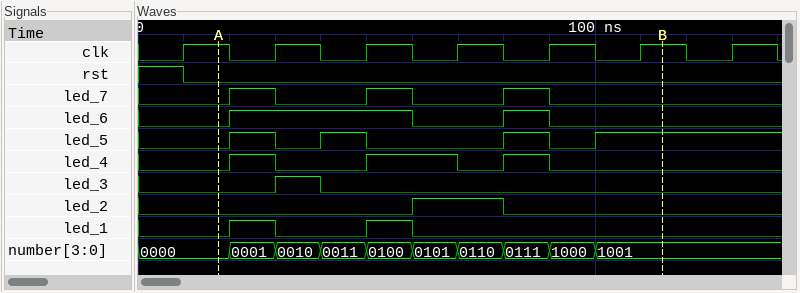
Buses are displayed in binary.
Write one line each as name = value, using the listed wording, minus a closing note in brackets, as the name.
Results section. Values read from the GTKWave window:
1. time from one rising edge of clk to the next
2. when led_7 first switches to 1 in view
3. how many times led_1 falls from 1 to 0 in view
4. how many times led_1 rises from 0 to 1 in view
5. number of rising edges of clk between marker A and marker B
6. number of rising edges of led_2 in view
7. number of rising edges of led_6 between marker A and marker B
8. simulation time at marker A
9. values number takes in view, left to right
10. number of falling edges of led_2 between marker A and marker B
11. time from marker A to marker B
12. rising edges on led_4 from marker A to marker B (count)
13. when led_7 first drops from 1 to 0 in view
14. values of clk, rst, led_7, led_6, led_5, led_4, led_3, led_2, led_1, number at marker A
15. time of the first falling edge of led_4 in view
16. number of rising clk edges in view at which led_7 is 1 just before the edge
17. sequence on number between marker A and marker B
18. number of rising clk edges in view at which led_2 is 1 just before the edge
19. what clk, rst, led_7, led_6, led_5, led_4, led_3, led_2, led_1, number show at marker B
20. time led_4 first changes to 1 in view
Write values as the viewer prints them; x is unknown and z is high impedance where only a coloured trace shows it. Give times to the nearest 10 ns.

time from one rising edge of clk to the next = 20 ns
when led_7 first switches to 1 in view = 20 ns
how many times led_1 falls from 1 to 0 in view = 2
how many times led_1 rises from 0 to 1 in view = 2
number of rising edges of clk between marker A and marker B = 5
number of rising edges of led_2 in view = 1
number of rising edges of led_6 between marker A and marker B = 2
simulation time at marker A = 20 ns
values number takes in view, left to right = 0000, 0001, 0010, 0011, 0100, 0101, 0110, 0111, 1000, 1001
number of falling edges of led_2 between marker A and marker B = 1
time from marker A to marker B = 100 ns
rising edges on led_4 from marker A to marker B = 3
when led_7 first drops from 1 to 0 in view = 30 ns
values of clk, rst, led_7, led_6, led_5, led_4, led_3, led_2, led_1, number at marker A = clk=1, rst=0, led_7=0, led_6=0, led_5=0, led_4=0, led_3=0, led_2=0, led_1=0, number=0000
time of the first falling edge of led_4 in view = 30 ns
number of rising clk edges in view at which led_7 is 1 just before the edge = 2
sequence on number between marker A and marker B = 0000, 0001, 0010, 0011, 0100, 0101, 0110, 0111, 1000, 1001
number of rising clk edges in view at which led_2 is 1 just before the edge = 1
what clk, rst, led_7, led_6, led_5, led_4, led_3, led_2, led_1, number show at marker B = clk=1, rst=0, led_7=0, led_6=0, led_5=1, led_4=0, led_3=0, led_2=0, led_1=0, number=1001
time led_4 first changes to 1 in view = 20 ns
